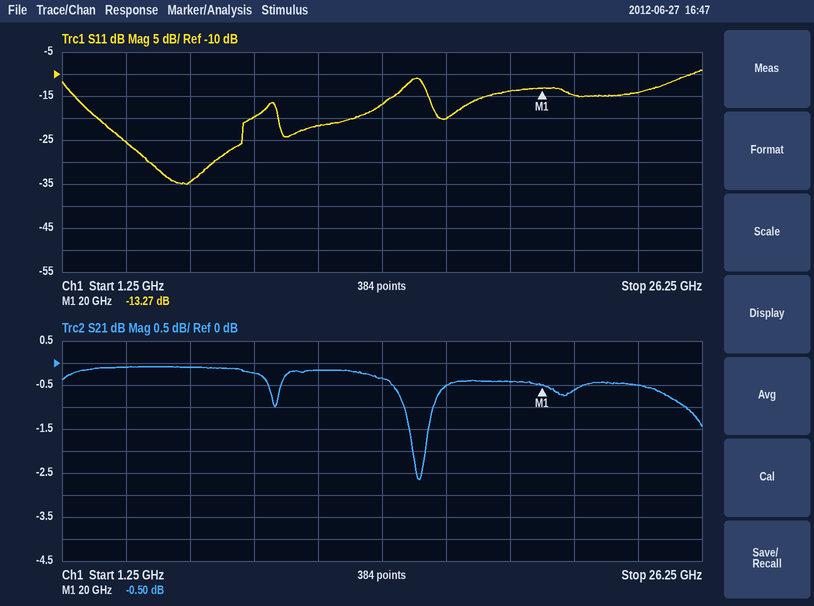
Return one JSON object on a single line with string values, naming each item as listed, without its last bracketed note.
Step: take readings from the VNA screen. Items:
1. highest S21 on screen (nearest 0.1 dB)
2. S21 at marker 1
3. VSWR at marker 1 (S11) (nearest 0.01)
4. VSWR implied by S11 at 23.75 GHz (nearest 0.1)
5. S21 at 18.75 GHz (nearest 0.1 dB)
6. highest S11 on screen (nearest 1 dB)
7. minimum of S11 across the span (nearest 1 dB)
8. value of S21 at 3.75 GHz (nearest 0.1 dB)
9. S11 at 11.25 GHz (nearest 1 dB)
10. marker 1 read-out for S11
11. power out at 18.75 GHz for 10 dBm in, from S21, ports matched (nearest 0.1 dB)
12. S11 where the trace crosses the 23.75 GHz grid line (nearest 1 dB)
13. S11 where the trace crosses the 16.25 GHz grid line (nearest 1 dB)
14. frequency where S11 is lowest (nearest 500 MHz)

{"highest S21 on screen": "-0.1 dB", "S21 at marker 1": "-0.50 dB", "VSWR at marker 1 (S11)": "1.55", "VSWR implied by S11 at 23.75 GHz": "1.5", "S21 at 18.75 GHz": "-0.4 dB", "highest S11 on screen": "-9 dB", "minimum of S11 across the span": "-35 dB", "value of S21 at 3.75 GHz": "-0.1 dB", "S11 at 11.25 GHz": "-22 dB", "marker 1 read-out for S11": "-13.27 dB", "power out at 18.75 GHz for 10 dBm in, from S21, ports matched": "9.6 dBm", "S11 where the trace crosses the 23.75 GHz grid line": "-14 dB", "S11 where the trace crosses the 16.25 GHz grid line": "-20 dB", "frequency where S11 is lowest": "6.0 GHz"}
